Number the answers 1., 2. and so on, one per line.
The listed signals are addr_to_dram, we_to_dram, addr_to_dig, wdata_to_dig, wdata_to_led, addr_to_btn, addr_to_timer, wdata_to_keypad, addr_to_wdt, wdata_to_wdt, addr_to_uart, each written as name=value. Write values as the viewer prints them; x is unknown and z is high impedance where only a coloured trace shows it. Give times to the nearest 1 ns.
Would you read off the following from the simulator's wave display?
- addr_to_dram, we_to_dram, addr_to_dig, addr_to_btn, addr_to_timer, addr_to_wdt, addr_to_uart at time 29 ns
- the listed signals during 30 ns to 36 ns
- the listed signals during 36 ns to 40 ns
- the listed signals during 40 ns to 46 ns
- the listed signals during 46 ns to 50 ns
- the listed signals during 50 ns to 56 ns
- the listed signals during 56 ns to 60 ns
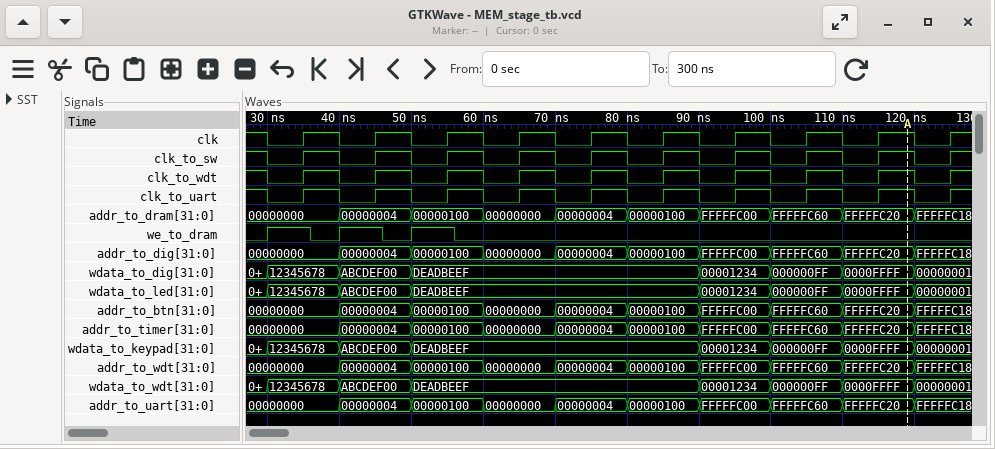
1. addr_to_dram=00000000, we_to_dram=0, addr_to_dig=00000000, addr_to_btn=00000000, addr_to_timer=00000000, addr_to_wdt=00000000, addr_to_uart=00000000
2. addr_to_dram=00000000, we_to_dram=1, addr_to_dig=00000000, wdata_to_dig=12345678, wdata_to_led=12345678, addr_to_btn=00000000, addr_to_timer=00000000, wdata_to_keypad=12345678, addr_to_wdt=00000000, wdata_to_wdt=12345678, addr_to_uart=00000000
3. addr_to_dram=00000000, we_to_dram=0, addr_to_dig=00000000, wdata_to_dig=12345678, wdata_to_led=12345678, addr_to_btn=00000000, addr_to_timer=00000000, wdata_to_keypad=12345678, addr_to_wdt=00000000, wdata_to_wdt=12345678, addr_to_uart=00000000
4. addr_to_dram=00000004, we_to_dram=1, addr_to_dig=00000004, wdata_to_dig=ABCDEF00, wdata_to_led=ABCDEF00, addr_to_btn=00000004, addr_to_timer=00000004, wdata_to_keypad=ABCDEF00, addr_to_wdt=00000004, wdata_to_wdt=ABCDEF00, addr_to_uart=00000004
5. addr_to_dram=00000004, we_to_dram=0, addr_to_dig=00000004, wdata_to_dig=ABCDEF00, wdata_to_led=ABCDEF00, addr_to_btn=00000004, addr_to_timer=00000004, wdata_to_keypad=ABCDEF00, addr_to_wdt=00000004, wdata_to_wdt=ABCDEF00, addr_to_uart=00000004
6. addr_to_dram=00000100, we_to_dram=1, addr_to_dig=00000100, wdata_to_dig=DEADBEEF, wdata_to_led=DEADBEEF, addr_to_btn=00000100, addr_to_timer=00000100, wdata_to_keypad=DEADBEEF, addr_to_wdt=00000100, wdata_to_wdt=DEADBEEF, addr_to_uart=00000100
7. addr_to_dram=00000100, we_to_dram=0, addr_to_dig=00000100, wdata_to_dig=DEADBEEF, wdata_to_led=DEADBEEF, addr_to_btn=00000100, addr_to_timer=00000100, wdata_to_keypad=DEADBEEF, addr_to_wdt=00000100, wdata_to_wdt=DEADBEEF, addr_to_uart=00000100
